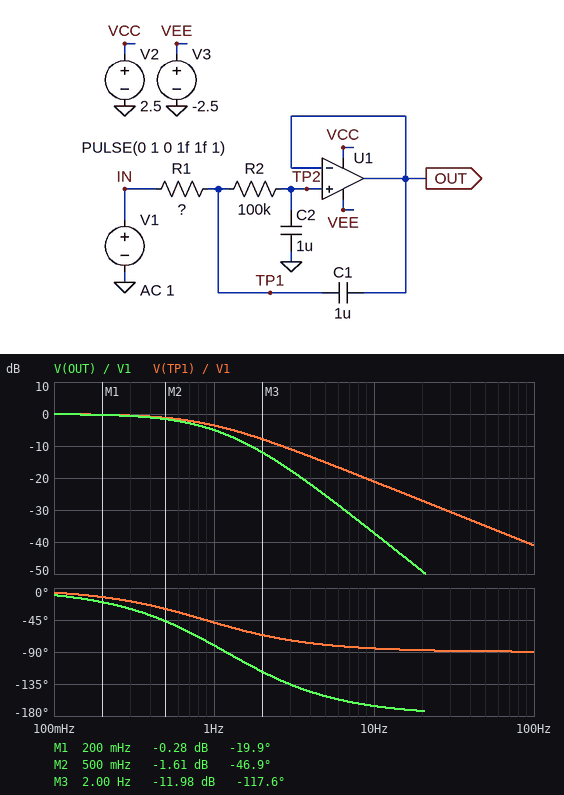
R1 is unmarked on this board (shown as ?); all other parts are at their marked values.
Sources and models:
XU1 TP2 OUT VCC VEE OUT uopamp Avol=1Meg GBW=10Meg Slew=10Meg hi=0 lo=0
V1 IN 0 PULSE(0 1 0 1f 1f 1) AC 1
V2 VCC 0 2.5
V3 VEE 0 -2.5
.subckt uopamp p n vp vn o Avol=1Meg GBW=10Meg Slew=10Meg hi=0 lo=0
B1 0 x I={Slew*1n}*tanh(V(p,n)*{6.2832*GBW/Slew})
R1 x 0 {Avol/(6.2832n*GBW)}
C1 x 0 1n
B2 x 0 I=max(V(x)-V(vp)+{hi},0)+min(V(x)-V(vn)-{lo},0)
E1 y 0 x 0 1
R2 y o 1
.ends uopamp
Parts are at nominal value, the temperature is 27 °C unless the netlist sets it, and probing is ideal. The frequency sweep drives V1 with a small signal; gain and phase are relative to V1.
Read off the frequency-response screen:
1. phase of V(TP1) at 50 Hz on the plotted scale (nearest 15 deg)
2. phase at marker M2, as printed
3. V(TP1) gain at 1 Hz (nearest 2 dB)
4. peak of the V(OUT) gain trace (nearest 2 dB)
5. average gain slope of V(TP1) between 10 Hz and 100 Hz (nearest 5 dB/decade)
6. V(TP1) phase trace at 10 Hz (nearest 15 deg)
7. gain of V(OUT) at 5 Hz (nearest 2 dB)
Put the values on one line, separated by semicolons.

-90 deg; -46.9 deg; -4 dB; 0 dB; -20 dB/decade; -90 deg; -26 dB
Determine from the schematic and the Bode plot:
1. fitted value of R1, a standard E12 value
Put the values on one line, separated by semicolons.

180 kΩ
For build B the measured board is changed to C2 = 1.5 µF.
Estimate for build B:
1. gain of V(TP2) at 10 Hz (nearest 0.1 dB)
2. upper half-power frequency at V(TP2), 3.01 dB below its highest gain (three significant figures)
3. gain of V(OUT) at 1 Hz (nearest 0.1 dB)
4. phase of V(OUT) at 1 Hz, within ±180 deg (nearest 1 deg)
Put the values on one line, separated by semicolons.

-40.7 dB; 445 mHz; -8.4 dB; -91 deg
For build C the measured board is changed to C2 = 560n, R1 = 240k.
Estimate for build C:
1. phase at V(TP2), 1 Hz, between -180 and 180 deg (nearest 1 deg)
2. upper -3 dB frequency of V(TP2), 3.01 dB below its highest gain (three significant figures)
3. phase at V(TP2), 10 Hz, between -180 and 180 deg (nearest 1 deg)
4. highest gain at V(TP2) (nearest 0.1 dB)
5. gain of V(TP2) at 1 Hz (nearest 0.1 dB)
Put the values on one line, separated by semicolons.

-69 deg; 1.16 Hz; -167 deg; 0 dB; -2.2 dB
